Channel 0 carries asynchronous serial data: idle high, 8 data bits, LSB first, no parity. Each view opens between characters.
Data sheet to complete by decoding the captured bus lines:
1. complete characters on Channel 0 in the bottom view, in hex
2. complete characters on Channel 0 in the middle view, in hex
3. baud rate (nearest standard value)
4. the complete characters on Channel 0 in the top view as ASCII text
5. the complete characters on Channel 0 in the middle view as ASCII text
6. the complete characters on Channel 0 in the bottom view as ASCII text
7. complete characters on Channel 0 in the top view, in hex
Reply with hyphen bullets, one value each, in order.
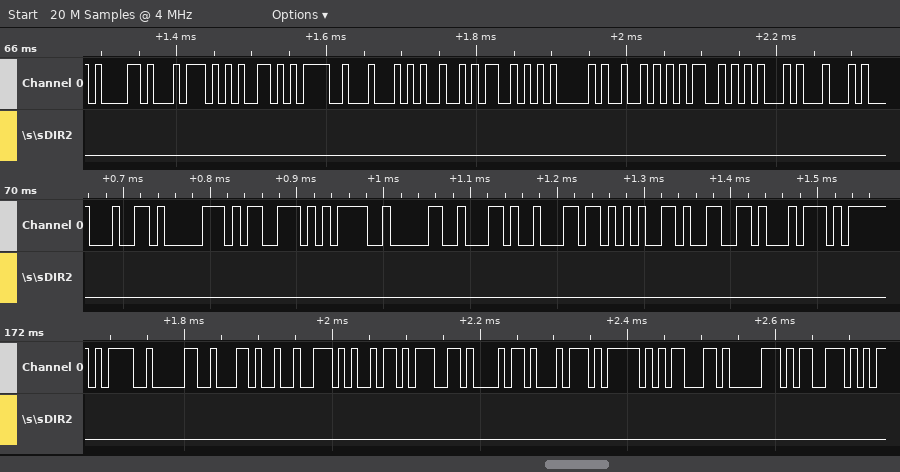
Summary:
- 3D, 30, 2C, 72, 69, 67, 68, 74, 5F, 63, 70, 73
- 64, 70, 73, 3D, 30, 2C, 6C, 65, 66, 74
- 115200 baud
- "ate=DISARMED"
- "dps=0,left"
- "=0,right_cps"
- 61, 74, 65, 3D, 44, 49, 53, 41, 52, 4D, 45, 44
